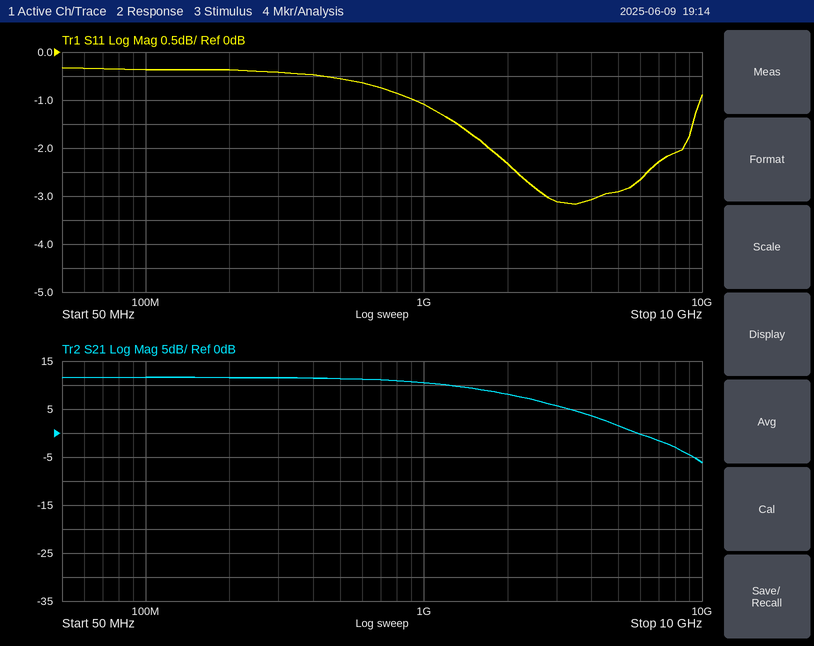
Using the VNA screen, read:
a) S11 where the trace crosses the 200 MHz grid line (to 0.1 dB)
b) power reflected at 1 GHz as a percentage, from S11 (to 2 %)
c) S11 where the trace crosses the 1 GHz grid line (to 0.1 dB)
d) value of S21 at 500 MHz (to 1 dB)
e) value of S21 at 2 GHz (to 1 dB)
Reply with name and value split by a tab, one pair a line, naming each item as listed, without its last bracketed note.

S11 where the trace crosses the 200 MHz grid line	-0.4 dB
power reflected at 1 GHz as a percentage, from S11	78 %
S11 where the trace crosses the 1 GHz grid line	-1.1 dB
value of S21 at 500 MHz	11 dB
value of S21 at 2 GHz	8 dB
